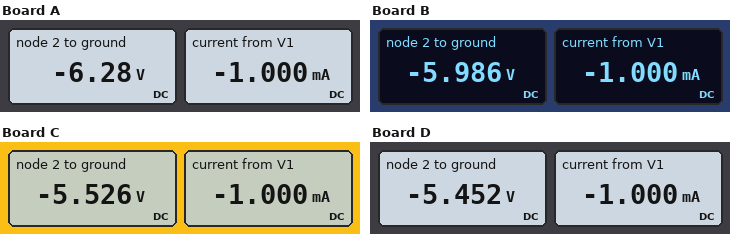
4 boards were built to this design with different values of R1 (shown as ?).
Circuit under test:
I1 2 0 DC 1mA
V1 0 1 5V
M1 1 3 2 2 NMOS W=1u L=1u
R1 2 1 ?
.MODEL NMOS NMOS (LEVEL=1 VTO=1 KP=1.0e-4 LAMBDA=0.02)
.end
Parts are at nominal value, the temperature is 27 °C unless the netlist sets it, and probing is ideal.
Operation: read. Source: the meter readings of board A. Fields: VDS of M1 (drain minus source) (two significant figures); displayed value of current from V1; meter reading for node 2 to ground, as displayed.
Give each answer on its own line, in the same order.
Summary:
1.3 V
-1.000 mA
-6.28 V
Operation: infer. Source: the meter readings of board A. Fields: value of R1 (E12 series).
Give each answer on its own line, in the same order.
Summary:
3.3 kΩ
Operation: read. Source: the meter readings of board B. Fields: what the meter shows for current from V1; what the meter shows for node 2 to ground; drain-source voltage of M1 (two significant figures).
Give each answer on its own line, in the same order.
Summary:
-1.000 mA
-5.986 V
990 mV
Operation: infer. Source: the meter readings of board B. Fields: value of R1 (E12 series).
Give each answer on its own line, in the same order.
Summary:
1.8 kΩ
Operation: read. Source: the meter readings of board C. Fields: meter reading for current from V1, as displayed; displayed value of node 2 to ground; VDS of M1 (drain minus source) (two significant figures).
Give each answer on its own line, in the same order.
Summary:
-1.000 mA
-5.526 V
530 mV
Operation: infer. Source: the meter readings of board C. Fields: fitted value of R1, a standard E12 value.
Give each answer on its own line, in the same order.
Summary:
680 Ω
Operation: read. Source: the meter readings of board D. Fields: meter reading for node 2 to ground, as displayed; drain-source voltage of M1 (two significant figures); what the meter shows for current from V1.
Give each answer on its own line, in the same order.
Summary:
-5.452 V
450 mV
-1.000 mA
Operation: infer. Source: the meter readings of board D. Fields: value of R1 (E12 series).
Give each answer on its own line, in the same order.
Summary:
560 Ω
